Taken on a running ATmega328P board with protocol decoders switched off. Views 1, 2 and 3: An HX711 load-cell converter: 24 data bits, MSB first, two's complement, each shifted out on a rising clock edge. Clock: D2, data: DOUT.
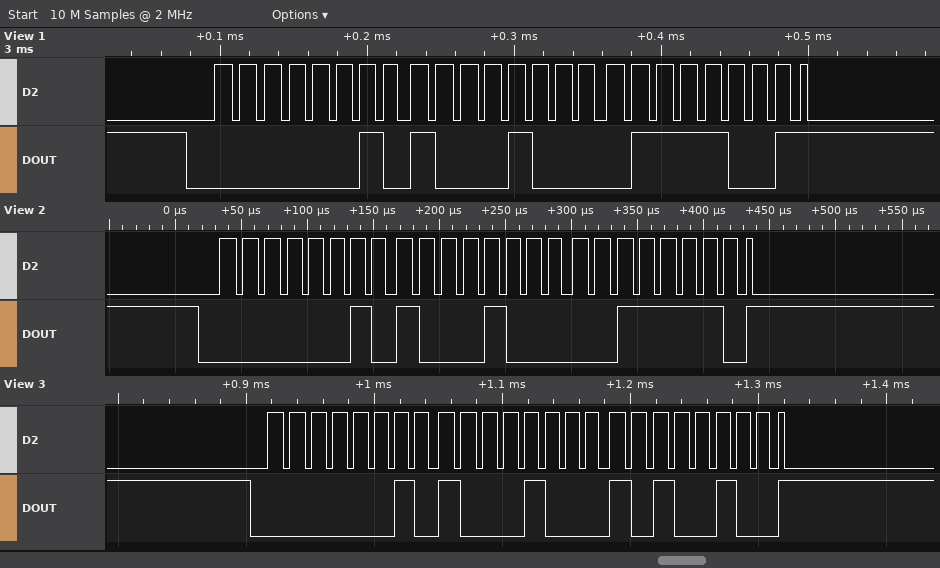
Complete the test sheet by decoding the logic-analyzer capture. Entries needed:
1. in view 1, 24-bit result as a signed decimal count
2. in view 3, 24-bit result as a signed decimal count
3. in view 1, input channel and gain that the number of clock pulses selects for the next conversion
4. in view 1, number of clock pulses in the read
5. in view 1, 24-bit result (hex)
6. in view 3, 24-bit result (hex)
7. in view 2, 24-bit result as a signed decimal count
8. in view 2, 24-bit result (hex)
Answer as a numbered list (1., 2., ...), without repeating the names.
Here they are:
1. 166009
2. 166052
3. channel A, gain 128
4. 25
5. 0x028879
6. 0x0288A4
7. 165950
8. 0x02883E
